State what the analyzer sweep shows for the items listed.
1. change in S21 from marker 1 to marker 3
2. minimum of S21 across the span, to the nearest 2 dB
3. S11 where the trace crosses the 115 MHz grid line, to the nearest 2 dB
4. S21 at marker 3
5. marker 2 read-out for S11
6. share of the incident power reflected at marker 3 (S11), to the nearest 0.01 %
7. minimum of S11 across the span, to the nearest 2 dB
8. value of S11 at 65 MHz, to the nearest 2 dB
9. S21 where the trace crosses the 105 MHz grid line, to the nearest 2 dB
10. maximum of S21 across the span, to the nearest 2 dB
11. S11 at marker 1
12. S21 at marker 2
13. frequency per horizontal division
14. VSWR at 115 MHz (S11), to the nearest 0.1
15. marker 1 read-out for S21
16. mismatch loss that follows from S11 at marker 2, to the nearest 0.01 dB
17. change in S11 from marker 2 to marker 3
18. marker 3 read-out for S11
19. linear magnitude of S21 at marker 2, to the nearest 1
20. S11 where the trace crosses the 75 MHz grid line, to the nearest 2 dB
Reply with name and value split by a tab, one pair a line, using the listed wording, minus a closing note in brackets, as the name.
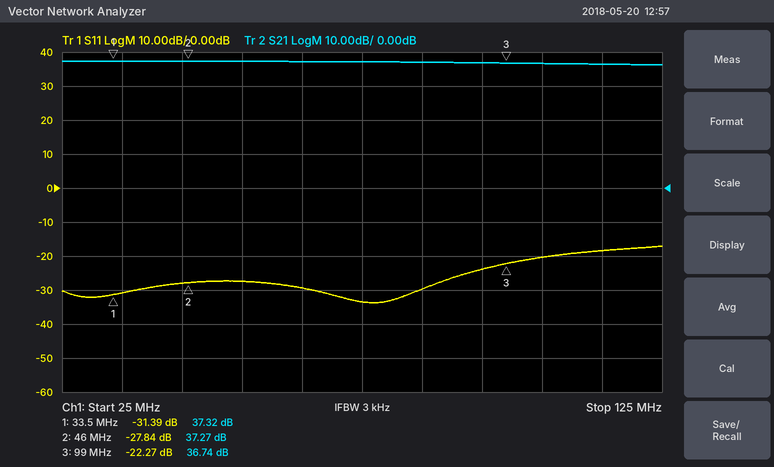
change in S21 from marker 1 to marker 3	-0.58 dB
minimum of S21 across the span, to the nearest 2 dB	36 dB
S11 where the trace crosses the 115 MHz grid line, to the nearest 2 dB	-18 dB
S21 at marker 3	36.74 dB
marker 2 read-out for S11	-27.84 dB
share of the incident power reflected at marker 3 (S11), to the nearest 0.01 %	0.59 %
minimum of S11 across the span, to the nearest 2 dB	-34 dB
value of S11 at 65 MHz, to the nearest 2 dB	-30 dB
S21 where the trace crosses the 105 MHz grid line, to the nearest 2 dB	36 dB
maximum of S21 across the span, to the nearest 2 dB	38 dB
S11 at marker 1	-31.39 dB
S21 at marker 2	37.27 dB
frequency per horizontal division	10 MHz
VSWR at 115 MHz (S11), to the nearest 0.1	1.3
marker 1 read-out for S21	37.32 dB
mismatch loss that follows from S11 at marker 2, to the nearest 0.01 dB	0.01 dB
change in S11 from marker 2 to marker 3	5.57 dB
marker 3 read-out for S11	-22.27 dB
linear magnitude of S21 at marker 2, to the nearest 1	73
S11 where the trace crosses the 75 MHz grid line, to the nearest 2 dB	-34 dB
